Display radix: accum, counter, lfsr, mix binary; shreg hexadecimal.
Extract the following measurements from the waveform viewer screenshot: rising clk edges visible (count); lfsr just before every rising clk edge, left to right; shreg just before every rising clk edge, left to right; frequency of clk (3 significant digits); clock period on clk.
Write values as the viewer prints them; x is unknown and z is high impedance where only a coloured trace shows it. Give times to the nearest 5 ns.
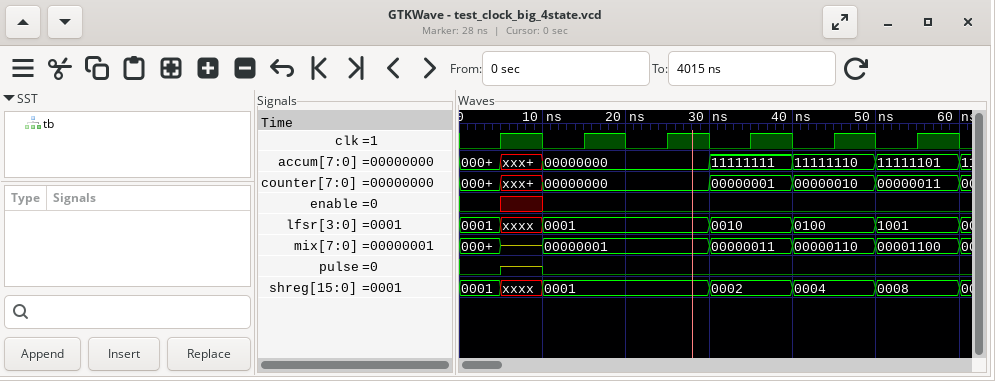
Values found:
6
0001, 0001, 0001, 0010, 0100, 1001
0001, 0001, 0001, 0002, 0004, 0008
100 MHz
10 ns
